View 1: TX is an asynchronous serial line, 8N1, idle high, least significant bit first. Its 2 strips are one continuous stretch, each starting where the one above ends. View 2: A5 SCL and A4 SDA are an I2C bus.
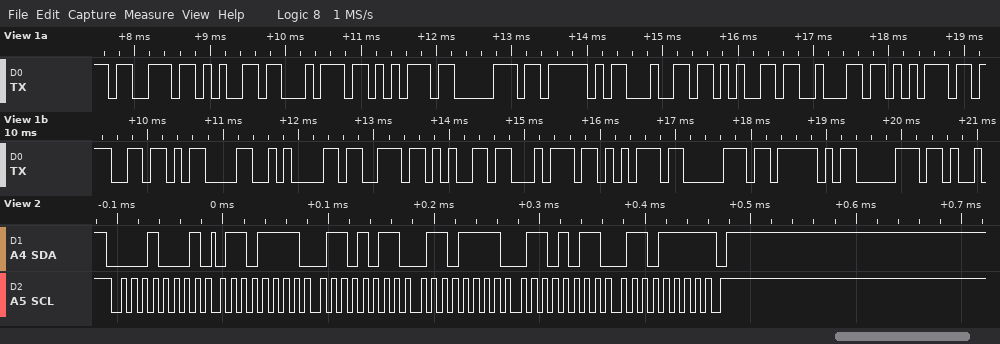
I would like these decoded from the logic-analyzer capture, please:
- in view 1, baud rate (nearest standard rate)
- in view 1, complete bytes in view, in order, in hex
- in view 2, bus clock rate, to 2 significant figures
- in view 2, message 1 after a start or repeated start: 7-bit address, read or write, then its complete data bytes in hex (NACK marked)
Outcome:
9600 baud
73 65 74 75 70 5F 64 65 62 75 67 0D 0A 73 65 74 75 70 5F 70
100 kHz
0x08 read: 6F 6B 6F 6B 6F NACK
